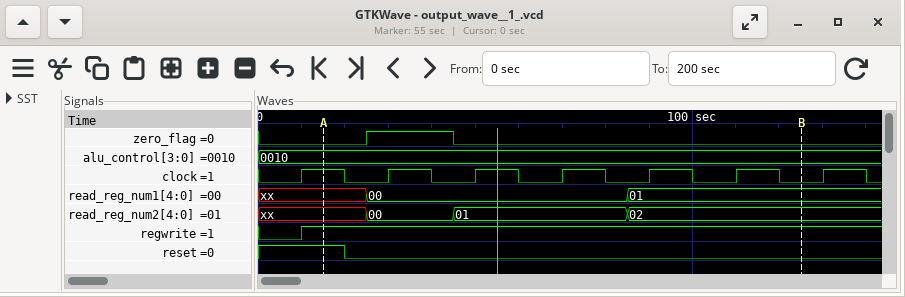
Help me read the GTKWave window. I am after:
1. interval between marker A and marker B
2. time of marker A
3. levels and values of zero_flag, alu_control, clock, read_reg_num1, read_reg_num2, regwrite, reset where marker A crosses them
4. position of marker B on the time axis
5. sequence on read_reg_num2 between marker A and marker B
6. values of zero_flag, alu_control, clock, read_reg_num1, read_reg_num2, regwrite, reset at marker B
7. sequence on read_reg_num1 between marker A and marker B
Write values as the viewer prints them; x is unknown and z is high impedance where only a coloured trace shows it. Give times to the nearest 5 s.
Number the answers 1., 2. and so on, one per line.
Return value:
1. 110 s
2. 15 s
3. zero_flag=0, alu_control=0010, clock=1, read_reg_num1=xx, read_reg_num2=xx, regwrite=1, reset=1
4. 125 s
5. xx, 00, 01, 02
6. zero_flag=0, alu_control=0010, clock=0, read_reg_num1=01, read_reg_num2=02, regwrite=1, reset=0
7. xx, 00, 01
